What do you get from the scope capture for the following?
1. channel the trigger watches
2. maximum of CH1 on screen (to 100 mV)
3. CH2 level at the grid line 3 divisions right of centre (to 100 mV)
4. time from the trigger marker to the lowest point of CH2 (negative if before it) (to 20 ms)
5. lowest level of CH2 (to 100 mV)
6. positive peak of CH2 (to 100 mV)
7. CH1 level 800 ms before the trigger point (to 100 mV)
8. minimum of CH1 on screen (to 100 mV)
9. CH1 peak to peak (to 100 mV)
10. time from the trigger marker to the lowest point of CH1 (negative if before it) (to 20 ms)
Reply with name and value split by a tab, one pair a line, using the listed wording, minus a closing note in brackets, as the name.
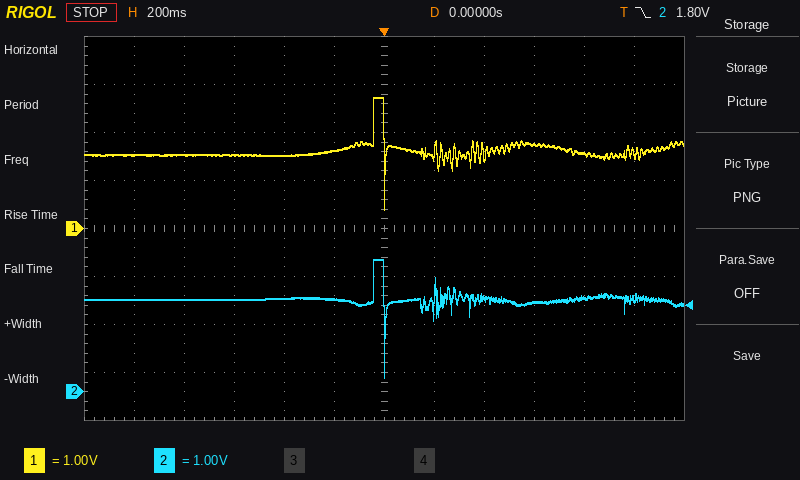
channel the trigger watches	CH2
maximum of CH1 on screen	2.7 V
CH2 level at the grid line 3 divisions right of centre	1.9 V
time from the trigger marker to the lowest point of CH2 (negative if before it)	0 ms
lowest level of CH2	300 mV
positive peak of CH2	2.8 V
CH1 level 800 ms before the trigger point	1.5 V
minimum of CH1 on screen	400 mV
CH1 peak to peak	2.3 V
time from the trigger marker to the lowest point of CH1 (negative if before it)	0 ms
